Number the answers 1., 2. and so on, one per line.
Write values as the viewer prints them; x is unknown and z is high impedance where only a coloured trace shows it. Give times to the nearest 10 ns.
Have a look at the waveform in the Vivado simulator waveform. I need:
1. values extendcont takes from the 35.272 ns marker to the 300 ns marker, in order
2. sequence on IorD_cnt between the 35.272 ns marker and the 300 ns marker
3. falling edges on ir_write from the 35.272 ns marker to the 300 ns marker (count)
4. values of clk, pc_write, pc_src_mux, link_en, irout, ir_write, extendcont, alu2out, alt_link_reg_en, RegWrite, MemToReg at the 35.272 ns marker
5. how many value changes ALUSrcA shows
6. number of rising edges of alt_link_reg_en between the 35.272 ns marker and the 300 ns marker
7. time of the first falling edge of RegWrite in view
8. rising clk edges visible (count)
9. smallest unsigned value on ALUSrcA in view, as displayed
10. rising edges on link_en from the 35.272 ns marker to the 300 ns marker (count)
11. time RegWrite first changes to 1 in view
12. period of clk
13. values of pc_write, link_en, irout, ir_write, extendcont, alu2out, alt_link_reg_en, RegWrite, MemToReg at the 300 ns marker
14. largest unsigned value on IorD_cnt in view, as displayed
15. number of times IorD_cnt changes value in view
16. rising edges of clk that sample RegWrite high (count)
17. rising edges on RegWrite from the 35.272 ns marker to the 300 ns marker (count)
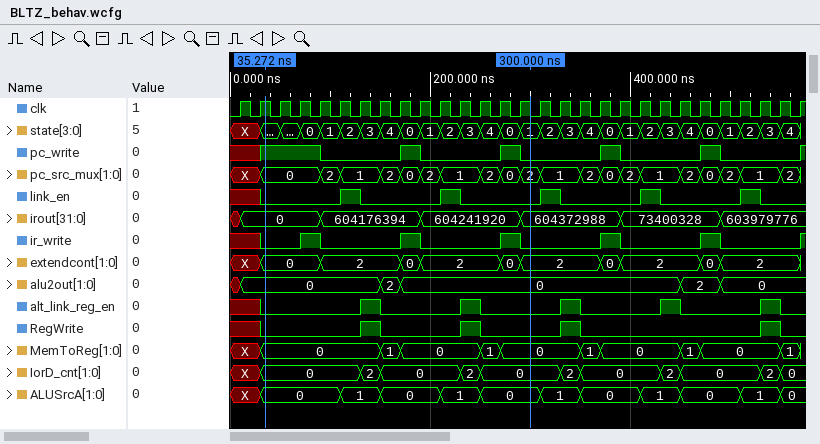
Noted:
1. 0, 2, 0, 2, 0, 2
2. 0, 2, 0, 2, 0
3. 3
4. clk=1, pc_write=1, pc_src_mux=0, link_en=0, irout=0, ir_write=0, extendcont=0, alu2out=0, alt_link_reg_en=0, RegWrite=0, MemToReg=0
5. 11
6. 2
7. 150 ns
8. 29
9. 0
10. 2
11. 130 ns
12. 20 ns
13. pc_write=0, link_en=0, irout=604372988, ir_write=0, extendcont=2, alu2out=0, alt_link_reg_en=0, RegWrite=0, MemToReg=0
14. 2
15. 11
16. 4
17. 2
